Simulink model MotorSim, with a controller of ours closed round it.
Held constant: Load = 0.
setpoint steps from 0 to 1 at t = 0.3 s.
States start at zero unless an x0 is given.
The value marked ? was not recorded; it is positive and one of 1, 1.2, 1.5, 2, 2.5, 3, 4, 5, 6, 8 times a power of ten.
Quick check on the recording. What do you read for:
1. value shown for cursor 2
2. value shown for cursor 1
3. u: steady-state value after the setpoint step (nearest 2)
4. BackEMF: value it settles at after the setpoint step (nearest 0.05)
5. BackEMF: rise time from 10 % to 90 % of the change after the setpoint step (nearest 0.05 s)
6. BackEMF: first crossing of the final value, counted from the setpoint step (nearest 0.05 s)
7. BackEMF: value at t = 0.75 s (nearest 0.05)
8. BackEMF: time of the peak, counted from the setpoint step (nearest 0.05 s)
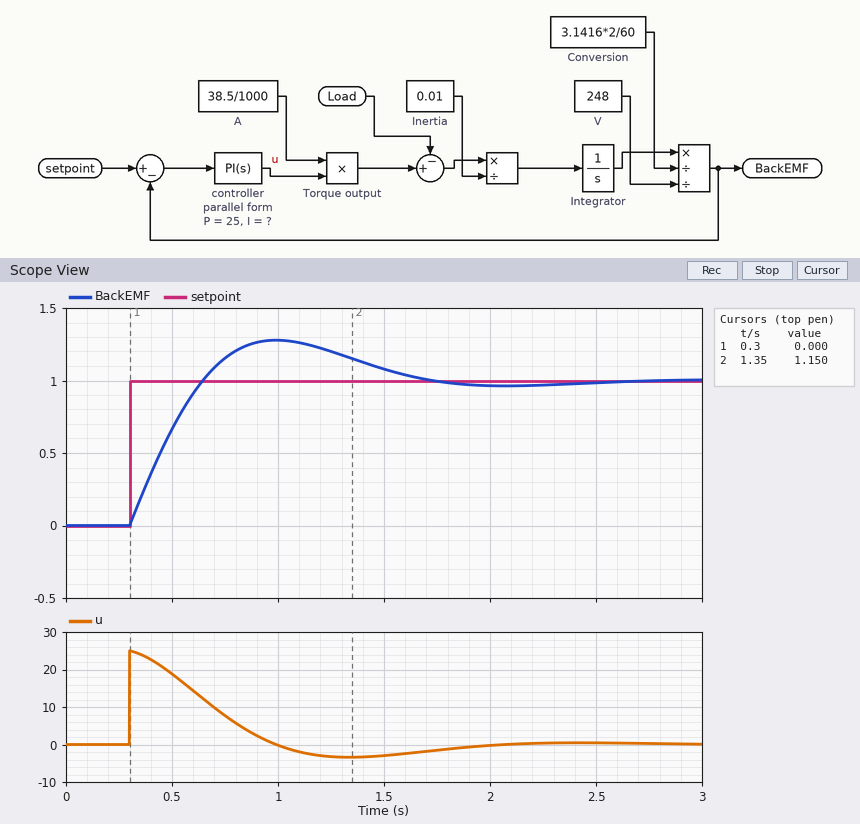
1.150
0.000
0
1.00
0.25 s
0.35 s
1.15
0.70 s
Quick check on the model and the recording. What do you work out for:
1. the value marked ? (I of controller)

80
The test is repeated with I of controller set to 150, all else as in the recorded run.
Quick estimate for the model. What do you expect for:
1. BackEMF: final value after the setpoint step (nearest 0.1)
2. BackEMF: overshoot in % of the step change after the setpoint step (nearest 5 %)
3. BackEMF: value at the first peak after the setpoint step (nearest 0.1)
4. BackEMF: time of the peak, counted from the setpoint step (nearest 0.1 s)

1.0
35 %
1.4
0.5 s
